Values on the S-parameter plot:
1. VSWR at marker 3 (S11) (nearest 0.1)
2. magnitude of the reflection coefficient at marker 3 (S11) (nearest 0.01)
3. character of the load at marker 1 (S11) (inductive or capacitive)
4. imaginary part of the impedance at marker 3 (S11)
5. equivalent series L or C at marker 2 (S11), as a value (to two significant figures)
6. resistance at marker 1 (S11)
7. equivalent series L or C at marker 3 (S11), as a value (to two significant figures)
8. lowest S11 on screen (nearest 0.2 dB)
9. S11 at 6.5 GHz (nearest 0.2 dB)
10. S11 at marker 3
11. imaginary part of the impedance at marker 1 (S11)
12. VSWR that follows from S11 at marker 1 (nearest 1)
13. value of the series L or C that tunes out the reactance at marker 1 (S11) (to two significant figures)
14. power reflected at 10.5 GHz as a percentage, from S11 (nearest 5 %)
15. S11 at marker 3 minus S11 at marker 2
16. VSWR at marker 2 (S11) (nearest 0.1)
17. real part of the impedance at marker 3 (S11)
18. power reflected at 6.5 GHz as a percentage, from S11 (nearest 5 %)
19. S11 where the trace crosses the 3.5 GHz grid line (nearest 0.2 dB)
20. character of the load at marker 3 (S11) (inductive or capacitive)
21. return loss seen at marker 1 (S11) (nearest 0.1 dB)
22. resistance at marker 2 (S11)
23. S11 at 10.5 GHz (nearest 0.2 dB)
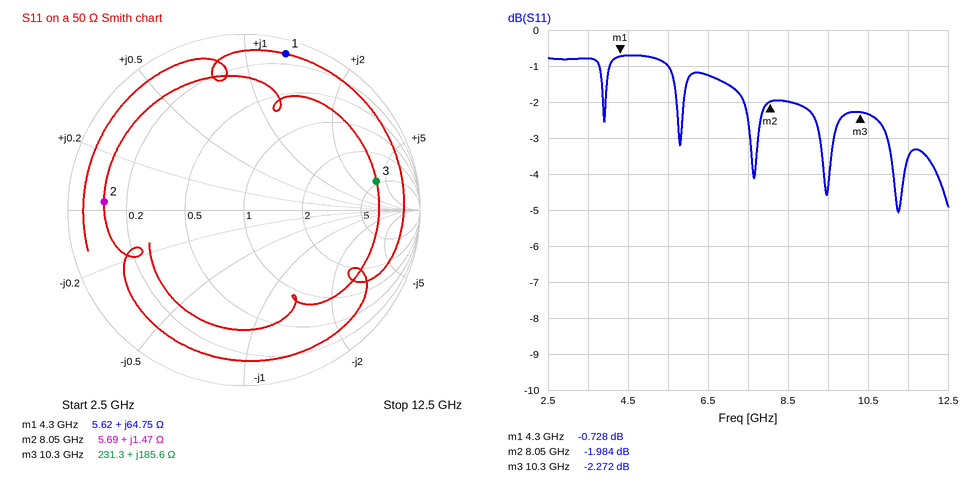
7.7
0.77
inductive
+185.6 Ω
29 pH
5.62 Ω
2.9 nH
-5.0 dB
-1.2 dB
-2.272 dB
+64.75 Ω
24
570 fF
60 %
-0.288 dB
8.8
231.3 Ω
75 %
-0.8 dB
inductive
0.7 dB
5.69 Ω
-2.4 dB
